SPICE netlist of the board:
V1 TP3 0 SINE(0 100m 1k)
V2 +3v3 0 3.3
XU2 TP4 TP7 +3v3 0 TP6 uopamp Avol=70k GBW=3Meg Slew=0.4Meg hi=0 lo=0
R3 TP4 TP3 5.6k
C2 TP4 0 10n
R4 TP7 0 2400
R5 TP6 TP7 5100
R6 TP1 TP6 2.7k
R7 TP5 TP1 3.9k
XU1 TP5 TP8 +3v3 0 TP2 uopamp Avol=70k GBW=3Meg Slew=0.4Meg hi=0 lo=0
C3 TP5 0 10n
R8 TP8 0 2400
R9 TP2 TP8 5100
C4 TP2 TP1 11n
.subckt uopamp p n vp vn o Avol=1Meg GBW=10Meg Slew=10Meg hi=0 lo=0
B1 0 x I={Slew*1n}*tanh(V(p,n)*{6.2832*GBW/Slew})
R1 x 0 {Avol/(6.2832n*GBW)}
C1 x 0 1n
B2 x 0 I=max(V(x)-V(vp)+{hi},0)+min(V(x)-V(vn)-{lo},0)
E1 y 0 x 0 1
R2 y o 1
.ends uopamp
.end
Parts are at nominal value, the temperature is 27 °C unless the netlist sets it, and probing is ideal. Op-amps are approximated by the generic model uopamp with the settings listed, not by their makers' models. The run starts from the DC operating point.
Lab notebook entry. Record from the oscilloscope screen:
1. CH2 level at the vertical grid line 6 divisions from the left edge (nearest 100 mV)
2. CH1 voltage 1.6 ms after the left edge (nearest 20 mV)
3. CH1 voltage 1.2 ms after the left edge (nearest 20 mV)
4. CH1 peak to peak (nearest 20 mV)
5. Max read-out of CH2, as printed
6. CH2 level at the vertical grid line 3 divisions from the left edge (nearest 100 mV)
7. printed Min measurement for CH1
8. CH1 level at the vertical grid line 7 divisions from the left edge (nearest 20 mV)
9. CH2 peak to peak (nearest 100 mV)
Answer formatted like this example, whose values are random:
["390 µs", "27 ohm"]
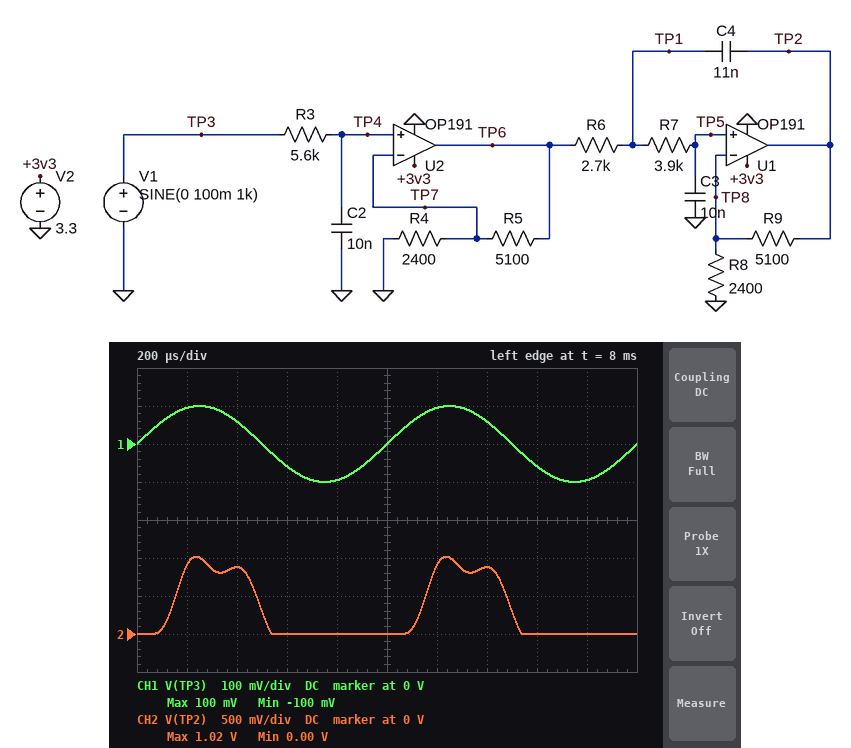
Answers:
["900 mV", "-60 mV", "100 mV", "200 mV", "1.02 V", "0 V", "-100 mV", "60 mV", "1.0 V"]
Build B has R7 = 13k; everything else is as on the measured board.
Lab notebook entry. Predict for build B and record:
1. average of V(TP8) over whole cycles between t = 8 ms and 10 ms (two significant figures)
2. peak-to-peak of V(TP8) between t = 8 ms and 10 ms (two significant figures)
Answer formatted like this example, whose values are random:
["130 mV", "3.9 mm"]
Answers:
["94 mV", "280 mV"]
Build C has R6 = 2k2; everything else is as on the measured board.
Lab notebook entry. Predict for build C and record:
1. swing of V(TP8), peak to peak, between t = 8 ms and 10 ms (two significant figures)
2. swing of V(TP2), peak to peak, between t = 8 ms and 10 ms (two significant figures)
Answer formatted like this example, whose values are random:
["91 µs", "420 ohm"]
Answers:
["290 mV", "920 mV"]
